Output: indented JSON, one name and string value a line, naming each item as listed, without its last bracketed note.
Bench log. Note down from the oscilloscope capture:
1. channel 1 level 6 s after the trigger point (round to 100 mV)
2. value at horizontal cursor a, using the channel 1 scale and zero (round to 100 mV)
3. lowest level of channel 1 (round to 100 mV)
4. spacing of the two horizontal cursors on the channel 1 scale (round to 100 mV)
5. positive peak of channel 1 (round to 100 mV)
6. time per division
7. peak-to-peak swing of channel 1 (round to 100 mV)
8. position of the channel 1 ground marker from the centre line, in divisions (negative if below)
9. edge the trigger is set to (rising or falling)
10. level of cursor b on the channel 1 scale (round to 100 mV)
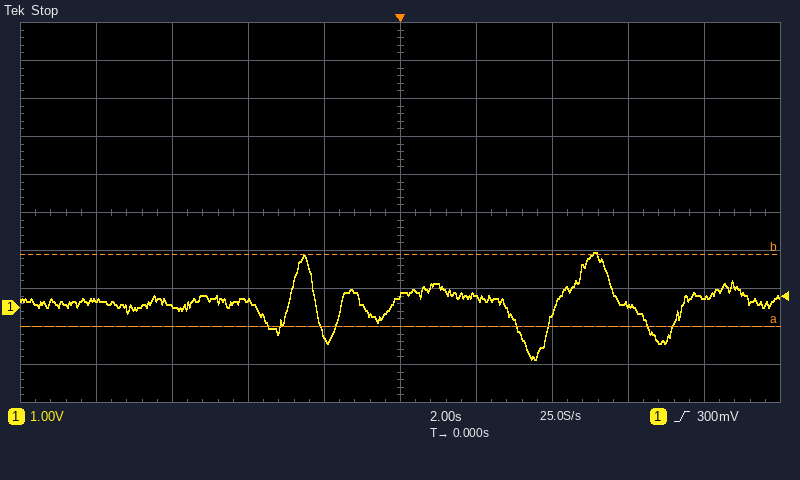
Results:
{
  "channel 1 level 6 s after the trigger point": "100 mV",
  "value at horizontal cursor a, using the channel 1 scale and zero": "-500 mV",
  "lowest level of channel 1": "-1.4 V",
  "spacing of the two horizontal cursors on the channel 1 scale": "1.9 V",
  "positive peak of channel 1": "1.4 V",
  "time per division": "2 s",
  "peak-to-peak swing of channel 1": "2.8 V",
  "position of the channel 1 ground marker from the centre line, in divisions": "-2.5 div",
  "edge the trigger is set to": "rising",
  "level of cursor b on the channel 1 scale": "1.4 V"
}
